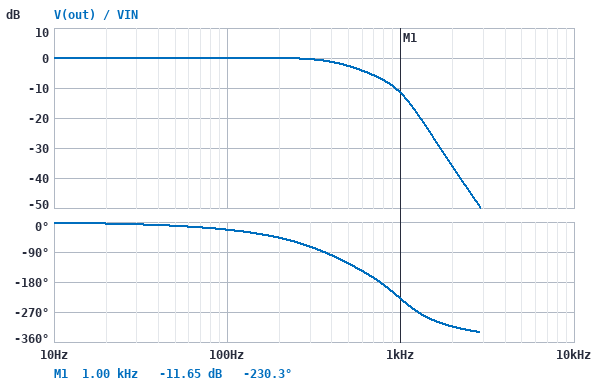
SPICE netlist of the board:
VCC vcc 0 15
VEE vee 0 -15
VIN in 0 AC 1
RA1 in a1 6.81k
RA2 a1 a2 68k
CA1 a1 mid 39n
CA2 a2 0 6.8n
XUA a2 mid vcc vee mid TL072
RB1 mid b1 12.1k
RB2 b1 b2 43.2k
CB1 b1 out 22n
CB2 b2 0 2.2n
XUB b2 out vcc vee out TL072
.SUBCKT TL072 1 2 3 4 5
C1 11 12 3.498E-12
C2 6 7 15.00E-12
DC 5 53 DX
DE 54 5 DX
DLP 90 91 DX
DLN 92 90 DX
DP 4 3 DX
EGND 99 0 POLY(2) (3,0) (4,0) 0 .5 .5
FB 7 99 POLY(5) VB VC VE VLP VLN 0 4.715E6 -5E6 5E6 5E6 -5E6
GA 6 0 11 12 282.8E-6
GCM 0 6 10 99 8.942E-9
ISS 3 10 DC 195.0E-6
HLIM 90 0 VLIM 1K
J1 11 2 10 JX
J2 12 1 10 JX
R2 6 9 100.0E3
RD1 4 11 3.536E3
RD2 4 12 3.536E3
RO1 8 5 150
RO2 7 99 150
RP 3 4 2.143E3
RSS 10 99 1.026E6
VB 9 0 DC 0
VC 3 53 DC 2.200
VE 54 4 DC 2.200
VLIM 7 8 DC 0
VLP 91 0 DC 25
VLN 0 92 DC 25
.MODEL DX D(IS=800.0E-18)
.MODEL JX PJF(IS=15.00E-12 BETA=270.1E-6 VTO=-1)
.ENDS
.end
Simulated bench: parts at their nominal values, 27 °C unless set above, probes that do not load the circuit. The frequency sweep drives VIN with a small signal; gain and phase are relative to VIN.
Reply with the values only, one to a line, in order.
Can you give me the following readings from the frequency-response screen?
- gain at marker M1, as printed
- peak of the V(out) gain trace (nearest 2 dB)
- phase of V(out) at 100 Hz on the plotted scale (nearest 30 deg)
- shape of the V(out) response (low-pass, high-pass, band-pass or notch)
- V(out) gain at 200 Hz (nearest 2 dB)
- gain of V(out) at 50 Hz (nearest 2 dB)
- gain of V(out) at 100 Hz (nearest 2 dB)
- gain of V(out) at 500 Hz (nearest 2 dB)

-11.65 dB
0 dB
-30 deg
low-pass
0 dB
0 dB
0 dB
-2 dB
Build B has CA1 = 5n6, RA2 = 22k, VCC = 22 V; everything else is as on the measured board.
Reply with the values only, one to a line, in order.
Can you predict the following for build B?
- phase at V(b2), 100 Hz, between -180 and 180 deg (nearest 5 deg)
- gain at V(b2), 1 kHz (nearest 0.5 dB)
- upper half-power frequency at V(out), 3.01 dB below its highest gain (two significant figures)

-10 deg
-1.0 dB
1.1 kHz
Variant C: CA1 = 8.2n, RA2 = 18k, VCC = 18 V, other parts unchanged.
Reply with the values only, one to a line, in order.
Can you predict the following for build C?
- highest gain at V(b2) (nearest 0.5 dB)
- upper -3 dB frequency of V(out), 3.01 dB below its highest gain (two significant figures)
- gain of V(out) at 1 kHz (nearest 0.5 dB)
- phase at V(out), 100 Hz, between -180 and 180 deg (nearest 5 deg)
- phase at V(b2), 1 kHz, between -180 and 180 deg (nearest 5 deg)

1.5 dB
1.1 kHz
0 dB
-10 deg
-145 deg
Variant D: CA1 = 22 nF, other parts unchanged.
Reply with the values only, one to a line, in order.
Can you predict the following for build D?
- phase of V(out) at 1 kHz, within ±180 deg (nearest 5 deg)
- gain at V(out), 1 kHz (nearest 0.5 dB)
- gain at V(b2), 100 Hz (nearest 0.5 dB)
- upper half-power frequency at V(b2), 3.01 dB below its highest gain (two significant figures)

150 deg
-9.0 dB
0 dB
530 Hz
